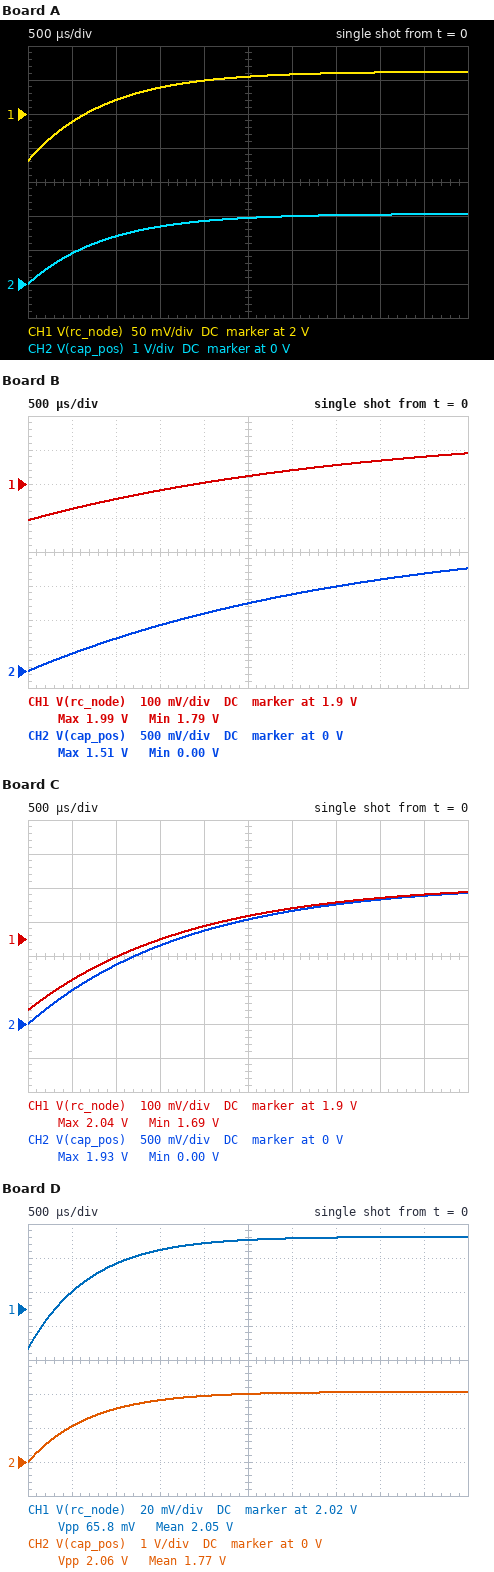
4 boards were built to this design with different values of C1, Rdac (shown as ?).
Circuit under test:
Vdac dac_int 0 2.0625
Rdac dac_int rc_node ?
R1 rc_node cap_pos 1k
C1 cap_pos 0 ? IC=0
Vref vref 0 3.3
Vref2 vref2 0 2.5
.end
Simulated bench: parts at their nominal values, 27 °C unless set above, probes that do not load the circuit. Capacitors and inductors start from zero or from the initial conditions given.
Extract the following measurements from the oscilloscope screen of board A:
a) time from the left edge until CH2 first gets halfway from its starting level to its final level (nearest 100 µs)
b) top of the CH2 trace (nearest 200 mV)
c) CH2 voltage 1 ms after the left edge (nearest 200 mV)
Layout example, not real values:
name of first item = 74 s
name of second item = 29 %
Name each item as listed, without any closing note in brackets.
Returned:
time from the left edge until CH2 first gets halfway from its starting level to its final level = 600 µs
top of the CH2 trace = 2.0 V
CH2 voltage 1 ms after the left edge = 1.4 V
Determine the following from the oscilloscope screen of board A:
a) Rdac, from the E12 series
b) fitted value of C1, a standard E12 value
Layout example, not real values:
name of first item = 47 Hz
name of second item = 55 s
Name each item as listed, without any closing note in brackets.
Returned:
Rdac, from the E12 series = 68 Ω
fitted value of C1, a standard E12 value = 820 nF
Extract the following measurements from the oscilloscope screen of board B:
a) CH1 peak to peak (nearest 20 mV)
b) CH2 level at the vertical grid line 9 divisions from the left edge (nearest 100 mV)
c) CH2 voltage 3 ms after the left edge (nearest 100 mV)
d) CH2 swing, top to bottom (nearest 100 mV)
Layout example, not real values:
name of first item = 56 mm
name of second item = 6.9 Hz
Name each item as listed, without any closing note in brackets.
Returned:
CH1 peak to peak = 200 mV
CH2 level at the vertical grid line 9 divisions from the left edge = 1.4 V
CH2 voltage 3 ms after the left edge = 1.1 V
CH2 swing, top to bottom = 1.5 V
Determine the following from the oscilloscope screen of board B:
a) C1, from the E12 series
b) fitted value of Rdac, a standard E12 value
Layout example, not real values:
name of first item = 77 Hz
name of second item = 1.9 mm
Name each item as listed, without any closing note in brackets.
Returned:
C1, from the E12 series = 3.3 µF
fitted value of Rdac, a standard E12 value = 150 Ω
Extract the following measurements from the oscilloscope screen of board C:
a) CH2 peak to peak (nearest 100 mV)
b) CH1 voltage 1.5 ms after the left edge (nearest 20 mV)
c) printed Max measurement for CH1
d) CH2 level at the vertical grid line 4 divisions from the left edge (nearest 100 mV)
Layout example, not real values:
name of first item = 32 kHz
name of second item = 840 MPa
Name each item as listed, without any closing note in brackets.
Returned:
CH2 peak to peak = 1.9 V
CH1 voltage 1.5 ms after the left edge = 1.90 V
printed Max measurement for CH1 = 2.04 V
CH2 level at the vertical grid line 4 divisions from the left edge = 1.4 V
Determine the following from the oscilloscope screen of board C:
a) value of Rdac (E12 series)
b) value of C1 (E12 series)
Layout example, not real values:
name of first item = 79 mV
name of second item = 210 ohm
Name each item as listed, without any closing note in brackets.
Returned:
value of Rdac = 220 Ω
value of C1 = 1.5 µF
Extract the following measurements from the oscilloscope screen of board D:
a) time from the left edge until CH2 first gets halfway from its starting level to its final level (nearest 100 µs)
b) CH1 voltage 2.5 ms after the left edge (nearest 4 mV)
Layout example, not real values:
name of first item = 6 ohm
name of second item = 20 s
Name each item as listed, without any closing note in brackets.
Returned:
time from the left edge until CH2 first gets halfway from its starting level to its final level = 500 µs
CH1 voltage 2.5 ms after the left edge = 2.060 V
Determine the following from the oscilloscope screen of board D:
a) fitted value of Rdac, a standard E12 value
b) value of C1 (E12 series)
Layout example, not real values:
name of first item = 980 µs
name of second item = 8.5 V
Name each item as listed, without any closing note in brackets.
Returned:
fitted value of Rdac, a standard E12 value = 33 Ω
value of C1 = 680 nF
